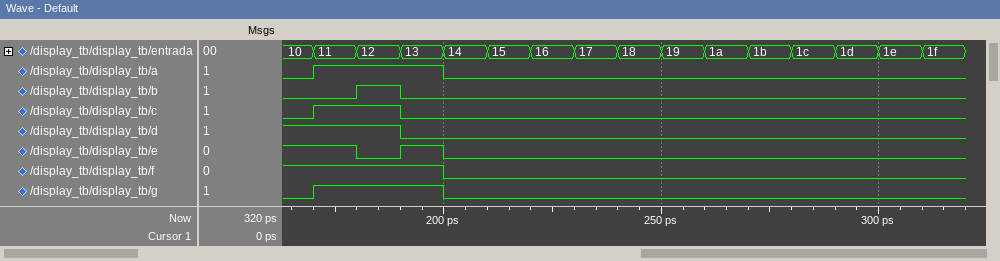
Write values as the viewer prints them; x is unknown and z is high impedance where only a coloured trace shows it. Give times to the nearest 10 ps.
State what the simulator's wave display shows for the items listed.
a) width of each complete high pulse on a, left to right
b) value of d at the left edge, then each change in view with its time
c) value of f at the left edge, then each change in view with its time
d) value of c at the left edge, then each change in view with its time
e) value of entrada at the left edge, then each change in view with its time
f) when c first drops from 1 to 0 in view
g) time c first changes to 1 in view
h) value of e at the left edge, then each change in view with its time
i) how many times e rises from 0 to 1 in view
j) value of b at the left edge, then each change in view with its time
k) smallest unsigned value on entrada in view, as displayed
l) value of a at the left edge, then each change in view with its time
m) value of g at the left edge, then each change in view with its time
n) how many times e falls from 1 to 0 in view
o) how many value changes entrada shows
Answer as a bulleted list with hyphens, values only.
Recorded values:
- 30 ps
- 1, 0 at 190 ps
- 1, 0 at 200 ps
- 0, 1 at 170 ps, 0 at 190 ps
- 10, 11 at 170 ps, 12 at 180 ps, 13 at 190 ps, 14 at 200 ps, 15 at 210 ps, 16 at 220 ps, 17 at 230 ps, 18 at 240 ps, 19 at 250 ps, 1a at 260 ps, 1b at 270 ps, 1c at 280 ps, 1d at 290 ps, 1e at 300 ps, 1f at 310 ps
- 190 ps
- 170 ps
- 1, 0 at 180 ps, 1 at 190 ps, 0 at 200 ps
- 1
- 0, 1 at 180 ps, 0 at 190 ps
- 10
- 0, 1 at 170 ps, 0 at 200 ps
- 0, 1 at 170 ps, 0 at 200 ps
- 2
- 15
